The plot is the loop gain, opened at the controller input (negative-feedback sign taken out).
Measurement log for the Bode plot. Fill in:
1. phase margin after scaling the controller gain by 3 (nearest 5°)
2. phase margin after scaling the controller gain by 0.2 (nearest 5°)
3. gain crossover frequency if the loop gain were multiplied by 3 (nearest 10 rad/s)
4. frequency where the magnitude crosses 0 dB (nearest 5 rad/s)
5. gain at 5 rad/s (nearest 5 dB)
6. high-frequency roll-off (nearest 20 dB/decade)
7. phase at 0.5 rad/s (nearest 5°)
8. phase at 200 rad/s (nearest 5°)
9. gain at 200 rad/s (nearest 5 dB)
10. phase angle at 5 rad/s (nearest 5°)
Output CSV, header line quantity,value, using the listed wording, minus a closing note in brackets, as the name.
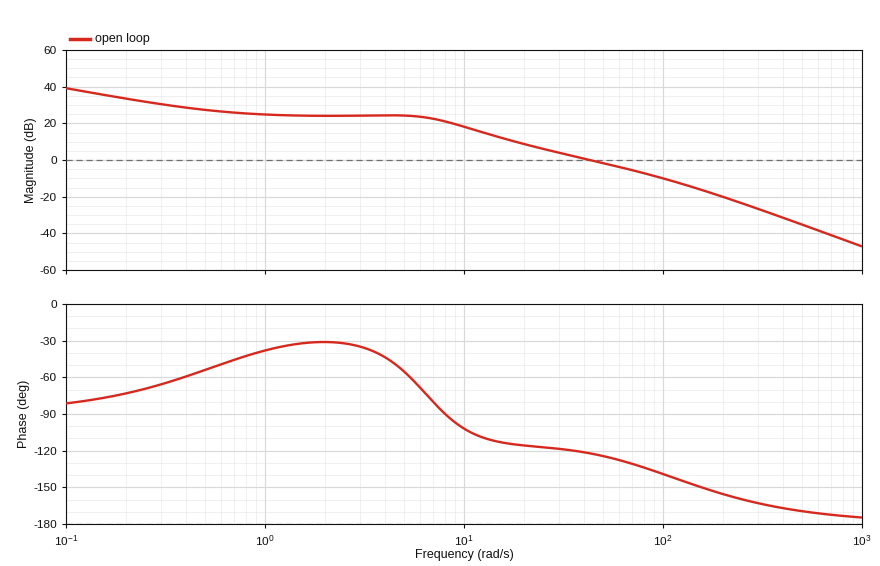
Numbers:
quantity,value
phase margin after scaling the controller gain by 3,40°
phase margin after scaling the controller gain by 0.2,70°
gain crossover frequency if the loop gain were multiplied by 3,100 rad/s
frequency where the magnitude crosses 0 dB,45 rad/s
gain at 5 rad/s,25 dB
high-frequency roll-off,-40 dB/decade
phase at 0.5 rad/s,-55°
phase at 200 rad/s,-155°
gain at 200 rad/s,-20 dB
phase angle at 5 rad/s,-55°
